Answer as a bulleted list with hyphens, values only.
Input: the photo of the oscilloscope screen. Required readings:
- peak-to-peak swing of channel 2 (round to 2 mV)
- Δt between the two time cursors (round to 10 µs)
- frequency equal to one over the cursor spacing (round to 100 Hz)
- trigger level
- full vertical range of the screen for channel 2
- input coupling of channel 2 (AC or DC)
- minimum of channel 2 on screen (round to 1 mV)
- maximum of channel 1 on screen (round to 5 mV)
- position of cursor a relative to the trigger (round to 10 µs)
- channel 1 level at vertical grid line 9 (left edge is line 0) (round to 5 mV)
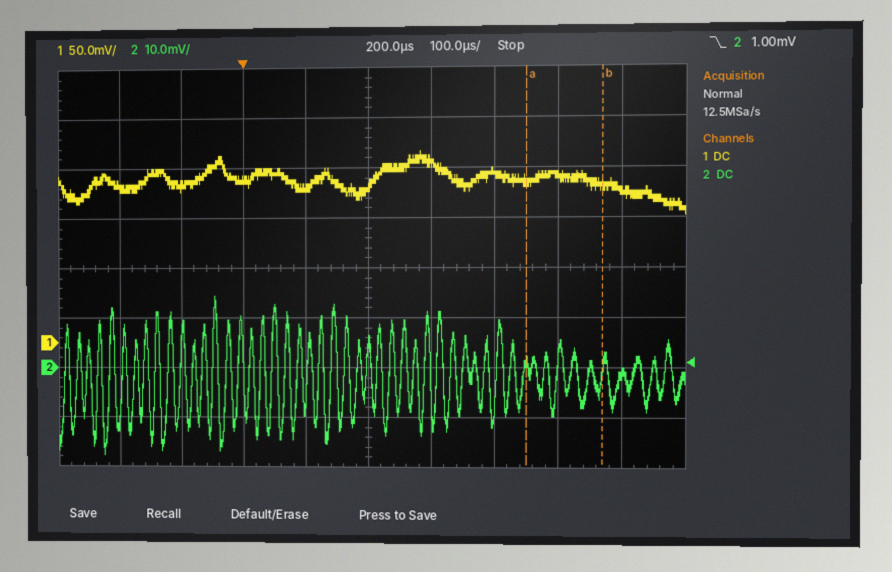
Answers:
- 32 mV
- 120 µs
- 8.3 kHz
- 1.00 mV
- 80 mV
- DC
- -18 mV
- 190 mV
- +450 µs
- 150 mV
